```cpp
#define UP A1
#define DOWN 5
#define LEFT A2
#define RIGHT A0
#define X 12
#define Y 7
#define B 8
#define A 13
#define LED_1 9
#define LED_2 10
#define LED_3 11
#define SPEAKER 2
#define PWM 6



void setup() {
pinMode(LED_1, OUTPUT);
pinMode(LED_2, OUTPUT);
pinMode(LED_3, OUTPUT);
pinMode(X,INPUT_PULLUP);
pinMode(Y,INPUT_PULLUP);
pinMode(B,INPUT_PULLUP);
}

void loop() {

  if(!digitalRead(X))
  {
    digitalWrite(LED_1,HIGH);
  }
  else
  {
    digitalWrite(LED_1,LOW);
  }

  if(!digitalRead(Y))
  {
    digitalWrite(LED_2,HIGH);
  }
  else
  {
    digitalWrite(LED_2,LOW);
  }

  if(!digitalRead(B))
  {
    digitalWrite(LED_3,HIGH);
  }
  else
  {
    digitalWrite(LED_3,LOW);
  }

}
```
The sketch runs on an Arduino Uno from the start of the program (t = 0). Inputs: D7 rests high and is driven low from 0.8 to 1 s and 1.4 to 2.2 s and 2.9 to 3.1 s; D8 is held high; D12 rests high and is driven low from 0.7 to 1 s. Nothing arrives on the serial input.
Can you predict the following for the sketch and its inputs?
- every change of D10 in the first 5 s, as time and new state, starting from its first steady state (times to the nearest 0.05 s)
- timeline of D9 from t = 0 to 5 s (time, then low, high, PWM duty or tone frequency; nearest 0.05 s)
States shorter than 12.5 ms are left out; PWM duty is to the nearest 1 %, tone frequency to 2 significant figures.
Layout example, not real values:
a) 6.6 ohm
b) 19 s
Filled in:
a) 0 s low; 0.8 s high; 1 s low; 1.4 s high; 2.2 s low; 2.9 s high; 3.1 s low
b) 0 s low; 0.7 s high; 1 s low
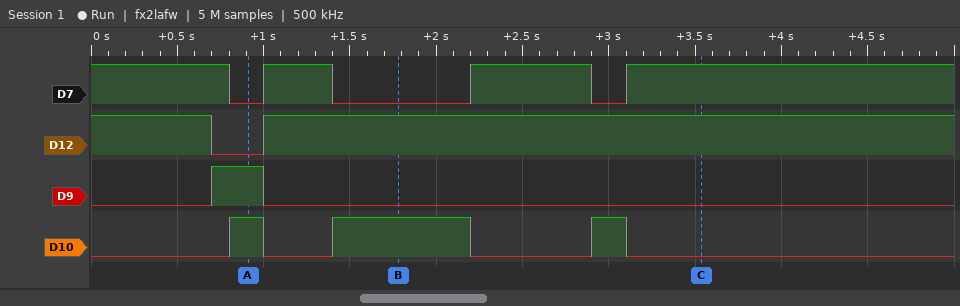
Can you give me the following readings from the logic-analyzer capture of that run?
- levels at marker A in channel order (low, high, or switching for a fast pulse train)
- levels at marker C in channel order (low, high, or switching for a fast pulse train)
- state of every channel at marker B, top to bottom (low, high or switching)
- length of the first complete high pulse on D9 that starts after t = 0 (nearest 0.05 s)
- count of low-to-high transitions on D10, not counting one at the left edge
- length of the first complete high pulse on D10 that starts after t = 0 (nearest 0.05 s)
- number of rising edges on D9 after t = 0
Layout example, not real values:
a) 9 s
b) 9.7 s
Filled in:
a) D7 low, D12 low, D9 high, D10 high
b) D7 high, D12 high, D9 low, D10 low
c) D7 low, D12 high, D9 low, D10 high
d) 0.30 s
e) 3
f) 0.20 s
g) 1
